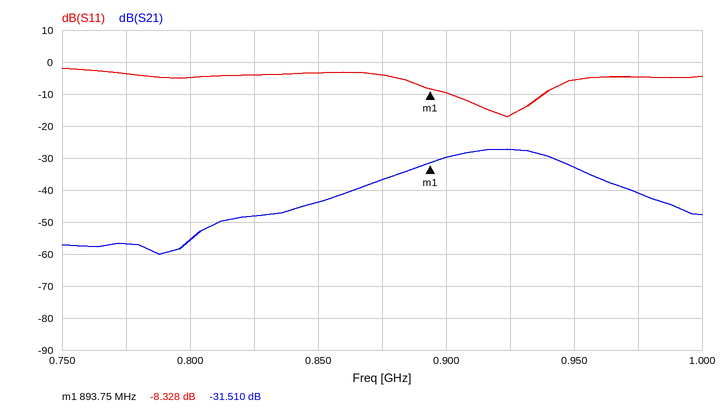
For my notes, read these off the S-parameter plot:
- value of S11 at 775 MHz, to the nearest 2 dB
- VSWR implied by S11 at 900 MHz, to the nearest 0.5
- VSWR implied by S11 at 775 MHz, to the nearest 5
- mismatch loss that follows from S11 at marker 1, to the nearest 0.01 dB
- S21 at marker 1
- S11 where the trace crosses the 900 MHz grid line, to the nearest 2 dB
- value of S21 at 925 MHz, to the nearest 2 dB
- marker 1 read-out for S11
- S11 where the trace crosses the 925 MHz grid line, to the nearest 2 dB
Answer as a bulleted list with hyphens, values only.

- -4 dB
- 2.0
- 5
- 0.69 dB
- -31.510 dB
- -10 dB
- -28 dB
- -8.328 dB
- -16 dB
